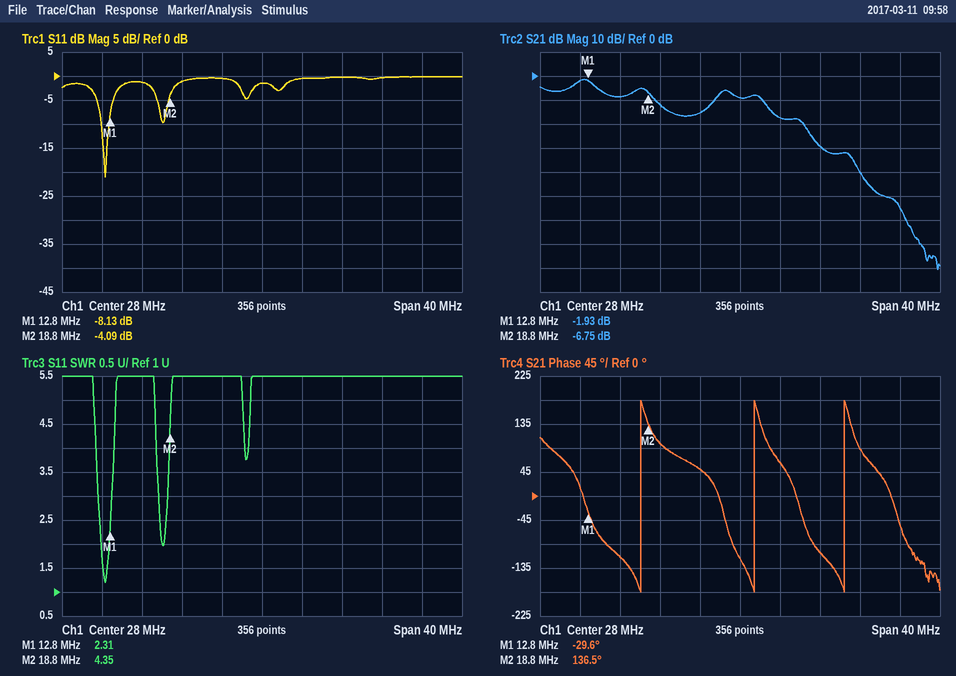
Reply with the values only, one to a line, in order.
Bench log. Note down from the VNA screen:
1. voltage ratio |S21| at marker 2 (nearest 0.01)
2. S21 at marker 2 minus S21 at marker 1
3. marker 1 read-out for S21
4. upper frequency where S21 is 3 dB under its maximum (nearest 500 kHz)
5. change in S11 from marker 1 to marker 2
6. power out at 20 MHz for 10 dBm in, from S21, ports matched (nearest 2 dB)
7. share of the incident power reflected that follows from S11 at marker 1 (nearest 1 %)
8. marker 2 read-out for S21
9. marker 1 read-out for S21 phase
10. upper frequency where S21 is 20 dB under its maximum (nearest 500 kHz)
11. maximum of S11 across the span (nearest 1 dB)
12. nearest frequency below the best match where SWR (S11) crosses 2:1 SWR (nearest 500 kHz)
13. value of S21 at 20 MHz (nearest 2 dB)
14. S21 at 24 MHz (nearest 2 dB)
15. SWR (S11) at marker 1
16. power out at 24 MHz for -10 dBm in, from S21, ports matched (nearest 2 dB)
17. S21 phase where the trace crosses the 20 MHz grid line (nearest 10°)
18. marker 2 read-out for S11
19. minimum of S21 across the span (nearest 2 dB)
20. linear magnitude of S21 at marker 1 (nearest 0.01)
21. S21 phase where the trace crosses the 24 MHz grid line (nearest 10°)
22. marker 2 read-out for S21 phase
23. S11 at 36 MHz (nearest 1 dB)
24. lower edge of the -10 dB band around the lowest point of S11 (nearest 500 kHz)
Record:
0.46
-4.82 dB
-1.93 dB
13.5 MHz
4.04 dB
-2 dBm
15 %
-6.75 dB
-29.6°
34.5 MHz
0 dB
12.0 MHz
-12 dB
-16 dB
2.31
-26 dBm
100°
-4.09 dB
-80 dB
0.80
50°
136.5°
0 dB
12.0 MHz
